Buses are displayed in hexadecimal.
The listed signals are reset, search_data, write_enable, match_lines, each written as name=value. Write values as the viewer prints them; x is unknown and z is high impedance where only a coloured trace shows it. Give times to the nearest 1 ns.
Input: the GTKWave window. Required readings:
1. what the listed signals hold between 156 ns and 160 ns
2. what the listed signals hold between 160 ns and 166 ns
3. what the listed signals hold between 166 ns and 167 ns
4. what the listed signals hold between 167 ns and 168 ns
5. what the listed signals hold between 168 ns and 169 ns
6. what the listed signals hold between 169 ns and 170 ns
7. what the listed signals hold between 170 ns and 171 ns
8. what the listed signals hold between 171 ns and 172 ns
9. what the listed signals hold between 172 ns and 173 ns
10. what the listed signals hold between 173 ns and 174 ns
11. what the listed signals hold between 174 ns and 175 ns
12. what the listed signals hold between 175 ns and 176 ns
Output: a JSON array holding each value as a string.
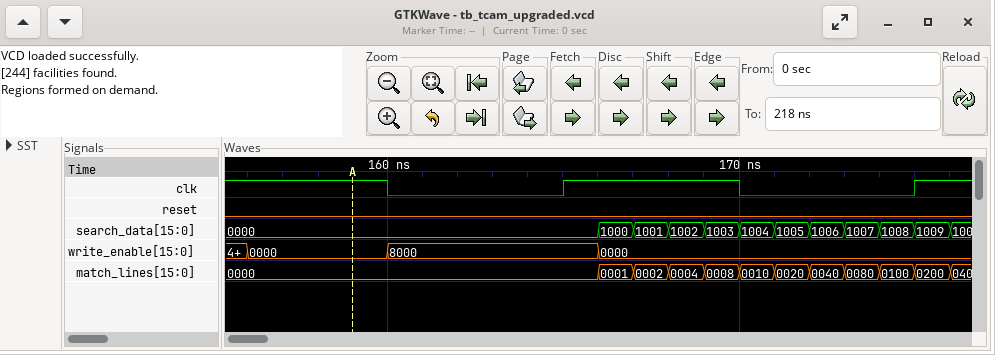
["reset=0, search_data=0000, write_enable=0000, match_lines=0000", "reset=0, search_data=0000, write_enable=8000, match_lines=0000", "reset=0, search_data=1000, write_enable=0000, match_lines=0001", "reset=0, search_data=1001, write_enable=0000, match_lines=0002", "reset=0, search_data=1002, write_enable=0000, match_lines=0004", "reset=0, search_data=1003, write_enable=0000, match_lines=0008", "reset=0, search_data=1004, write_enable=0000, match_lines=0010", "reset=0, search_data=1005, write_enable=0000, match_lines=0020", "reset=0, search_data=1006, write_enable=0000, match_lines=0040", "reset=0, search_data=1007, write_enable=0000, match_lines=0080", "reset=0, search_data=1008, write_enable=0000, match_lines=0100", "reset=0, search_data=1009, write_enable=0000, match_lines=0200"]
